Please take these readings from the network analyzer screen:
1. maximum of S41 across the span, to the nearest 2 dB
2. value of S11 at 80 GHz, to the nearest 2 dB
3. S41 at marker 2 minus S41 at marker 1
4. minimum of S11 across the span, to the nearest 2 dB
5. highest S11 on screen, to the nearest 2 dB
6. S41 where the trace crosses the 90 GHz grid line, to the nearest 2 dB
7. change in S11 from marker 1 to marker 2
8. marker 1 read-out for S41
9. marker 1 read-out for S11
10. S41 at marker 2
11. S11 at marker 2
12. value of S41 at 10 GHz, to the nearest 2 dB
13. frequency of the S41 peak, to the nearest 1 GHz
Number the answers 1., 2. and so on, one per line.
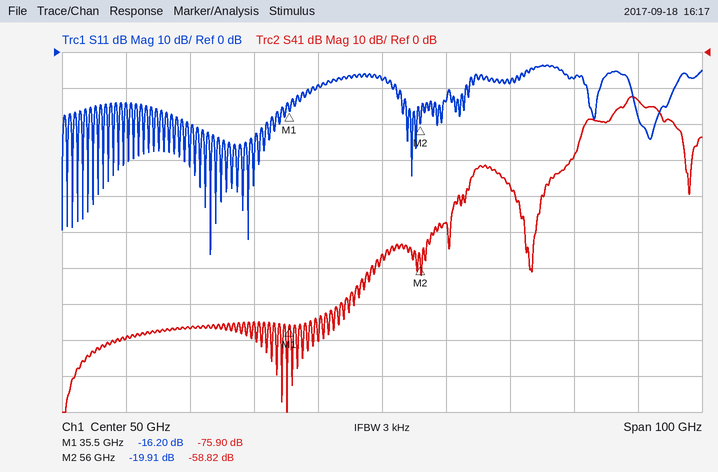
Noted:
1. -12 dB
2. -8 dB
3. 17.08 dB
4. -56 dB
5. -4 dB
6. -14 dB
7. -3.71 dB
8. -75.90 dB
9. -16.20 dB
10. -58.82 dB
11. -19.91 dB
12. -80 dB
13. 89 GHz
